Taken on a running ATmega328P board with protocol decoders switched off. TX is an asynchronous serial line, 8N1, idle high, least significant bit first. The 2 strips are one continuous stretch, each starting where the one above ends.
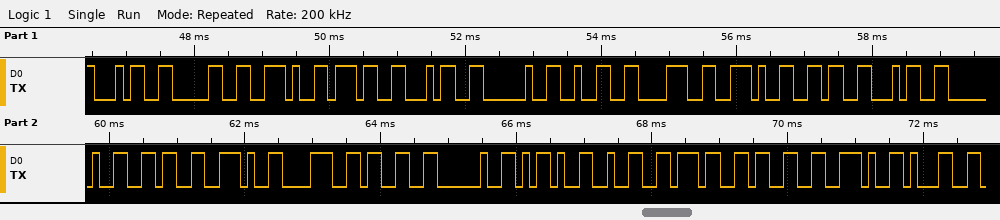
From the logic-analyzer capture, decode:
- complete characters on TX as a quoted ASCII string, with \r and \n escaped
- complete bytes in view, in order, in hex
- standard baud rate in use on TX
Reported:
"40.74 28.64 6.83 -273.1"
34 30 2E 37 34 20 32 38 2E 36 34 20 36 2E 38 33 20 2D 32 37 33 2E 31
9600 baud
